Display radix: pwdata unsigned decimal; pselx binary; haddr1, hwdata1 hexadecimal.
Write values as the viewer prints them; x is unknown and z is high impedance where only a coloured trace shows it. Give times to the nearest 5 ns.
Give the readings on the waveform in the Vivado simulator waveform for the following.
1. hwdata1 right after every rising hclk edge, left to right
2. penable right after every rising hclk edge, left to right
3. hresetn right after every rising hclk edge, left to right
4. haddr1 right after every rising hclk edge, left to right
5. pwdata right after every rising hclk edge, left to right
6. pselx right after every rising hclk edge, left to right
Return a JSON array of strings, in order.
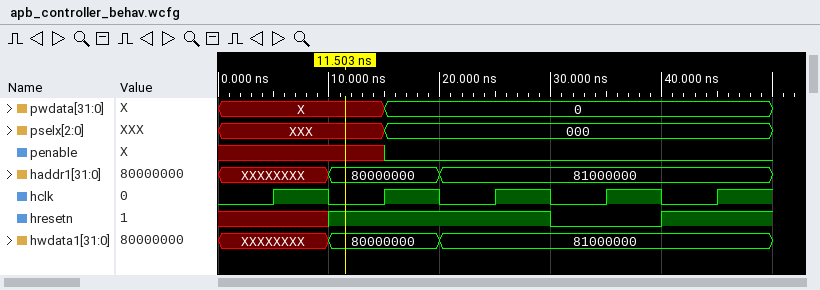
["XXXXXXXX, 80000000, 81000000, 81000000, 81000000", "x 0 0 0 0", "x 1 1 0 1", "XXXXXXXX, 80000000, 81000000, 81000000, 81000000", "X, 0, 0, 0, 0", "XXX, 000, 000, 000, 000"]
